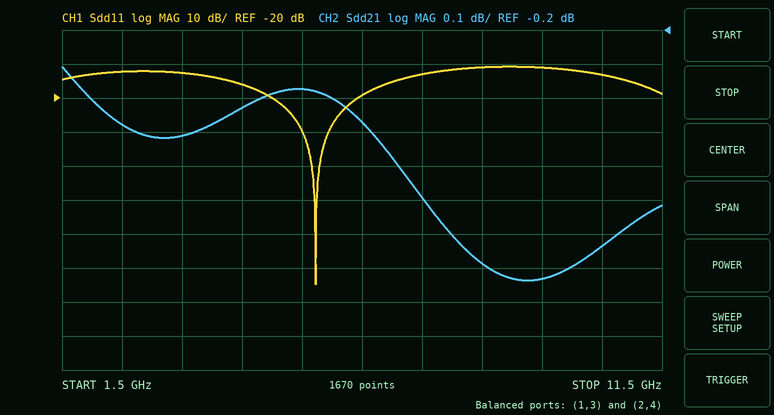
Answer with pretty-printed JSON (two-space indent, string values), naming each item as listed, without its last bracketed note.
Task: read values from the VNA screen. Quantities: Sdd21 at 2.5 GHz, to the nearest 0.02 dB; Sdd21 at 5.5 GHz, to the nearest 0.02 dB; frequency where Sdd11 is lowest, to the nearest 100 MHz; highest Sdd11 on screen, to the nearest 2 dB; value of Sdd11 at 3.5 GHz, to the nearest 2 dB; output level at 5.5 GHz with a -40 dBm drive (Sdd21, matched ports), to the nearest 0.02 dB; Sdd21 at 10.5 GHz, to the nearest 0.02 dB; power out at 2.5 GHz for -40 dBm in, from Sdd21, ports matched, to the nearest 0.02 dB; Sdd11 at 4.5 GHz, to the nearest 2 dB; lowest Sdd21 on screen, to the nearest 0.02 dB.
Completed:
{
  "Sdd21 at 2.5 GHz, to the nearest 0.02 dB": "-0.48 dB",
  "Sdd21 at 5.5 GHz, to the nearest 0.02 dB": "-0.38 dB",
  "frequency where Sdd11 is lowest, to the nearest 100 MHz": "5.7 GHz",
  "highest Sdd11 on screen, to the nearest 2 dB": "-10 dB",
  "value of Sdd11 at 3.5 GHz, to the nearest 2 dB": "-12 dB",
  "output level at 5.5 GHz with a -40 dBm drive (Sdd21, matched ports), to the nearest 0.02 dB": "-40.38 dBm",
  "Sdd21 at 10.5 GHz, to the nearest 0.02 dB": "-0.84 dB",
  "power out at 2.5 GHz for -40 dBm in, from Sdd21, ports matched, to the nearest 0.02 dB": "-40.48 dBm",
  "Sdd11 at 4.5 GHz, to the nearest 2 dB": "-16 dB",
  "lowest Sdd21 on screen, to the nearest 0.02 dB": "-0.94 dB"
}
